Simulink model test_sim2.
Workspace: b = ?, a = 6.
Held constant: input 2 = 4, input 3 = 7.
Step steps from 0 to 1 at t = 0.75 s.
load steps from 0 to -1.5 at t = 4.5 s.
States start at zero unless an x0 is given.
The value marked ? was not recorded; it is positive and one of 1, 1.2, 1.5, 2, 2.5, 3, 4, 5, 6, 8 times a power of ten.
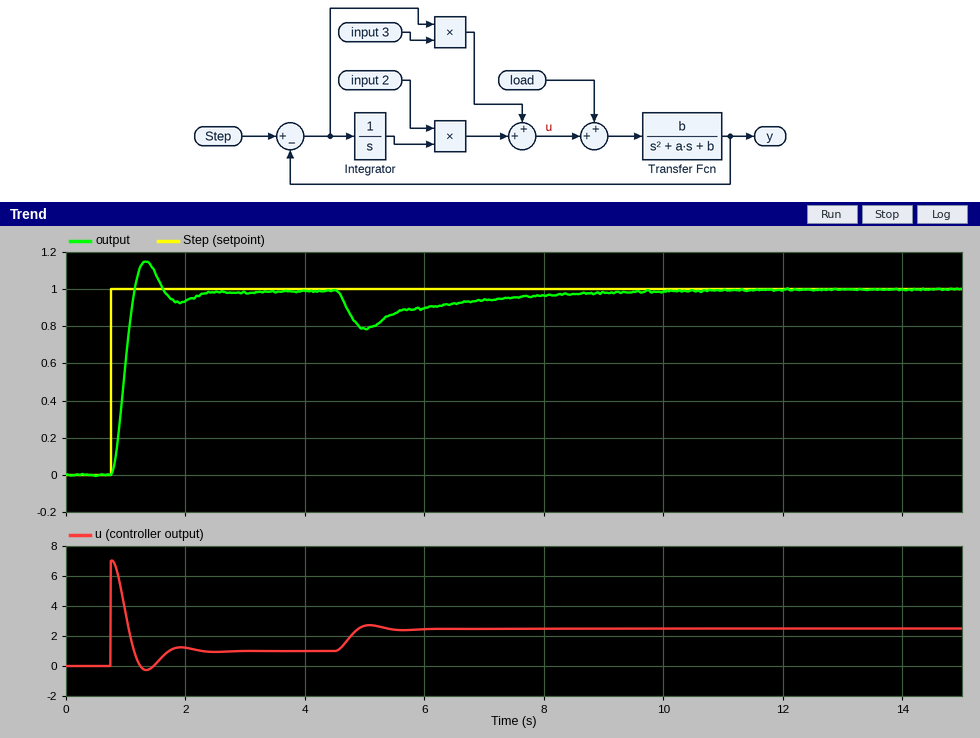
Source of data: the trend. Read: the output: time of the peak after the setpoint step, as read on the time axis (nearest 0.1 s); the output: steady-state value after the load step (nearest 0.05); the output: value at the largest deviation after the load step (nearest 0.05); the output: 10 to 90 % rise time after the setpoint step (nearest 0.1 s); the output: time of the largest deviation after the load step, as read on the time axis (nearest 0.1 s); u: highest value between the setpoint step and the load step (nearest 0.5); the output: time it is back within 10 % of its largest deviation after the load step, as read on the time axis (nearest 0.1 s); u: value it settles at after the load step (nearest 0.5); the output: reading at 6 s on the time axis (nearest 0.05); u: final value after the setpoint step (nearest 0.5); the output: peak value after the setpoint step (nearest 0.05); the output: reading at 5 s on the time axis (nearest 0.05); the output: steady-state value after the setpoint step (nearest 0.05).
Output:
1.3 s
1.00
0.80
0.3 s
5.0 s
7.0
8.9 s
2.5
0.90
1.0
1.15
0.80
1.00
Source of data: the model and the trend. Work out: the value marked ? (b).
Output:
5
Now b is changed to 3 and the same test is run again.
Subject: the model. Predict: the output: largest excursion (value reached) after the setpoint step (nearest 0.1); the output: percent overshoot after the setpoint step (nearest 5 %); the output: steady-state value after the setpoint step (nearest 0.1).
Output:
1.1
10 %
1.0
